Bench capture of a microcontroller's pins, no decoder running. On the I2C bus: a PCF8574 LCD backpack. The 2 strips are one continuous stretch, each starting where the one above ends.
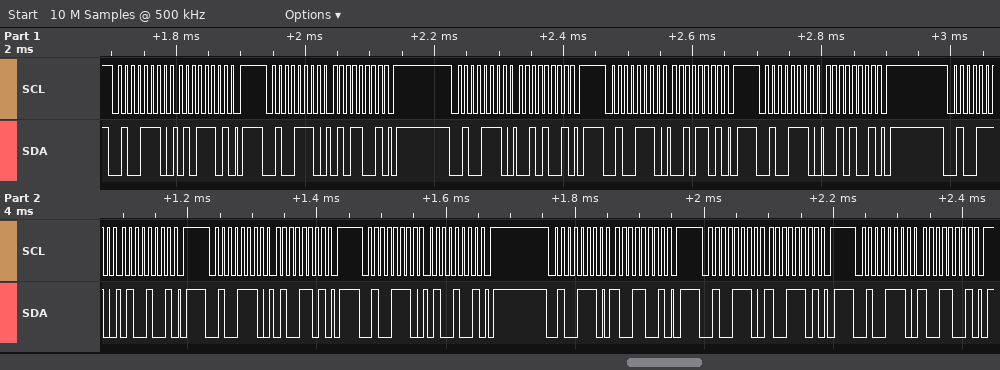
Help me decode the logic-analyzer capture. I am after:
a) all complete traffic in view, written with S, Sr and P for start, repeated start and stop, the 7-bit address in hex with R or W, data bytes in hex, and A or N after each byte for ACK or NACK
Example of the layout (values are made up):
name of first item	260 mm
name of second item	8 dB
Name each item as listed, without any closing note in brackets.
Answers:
all complete traffic in view, written with S, Sr and P for start, repeated start and stop, the 7-bit address in hex with R or W, data bytes in hex, and A or N after each byte for ACK or NACK	S 27W A 5D A P S 27W A 59 A P S 27W A 29 A P S 27W A 2D A P S 27W A 29 A P S 27W A 49 A P S 27W A 4D A P S 27W A 49 A P S 27W A 99 A P S 27W A 9D A P S 27W A 99 A P
